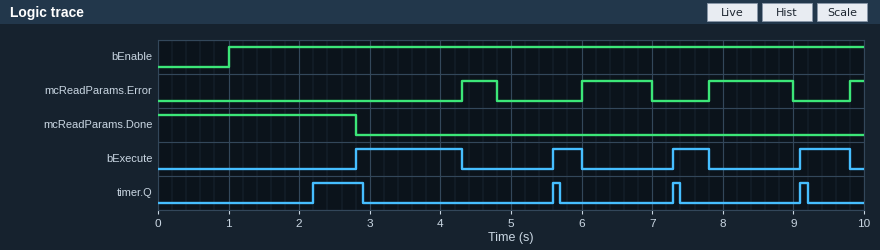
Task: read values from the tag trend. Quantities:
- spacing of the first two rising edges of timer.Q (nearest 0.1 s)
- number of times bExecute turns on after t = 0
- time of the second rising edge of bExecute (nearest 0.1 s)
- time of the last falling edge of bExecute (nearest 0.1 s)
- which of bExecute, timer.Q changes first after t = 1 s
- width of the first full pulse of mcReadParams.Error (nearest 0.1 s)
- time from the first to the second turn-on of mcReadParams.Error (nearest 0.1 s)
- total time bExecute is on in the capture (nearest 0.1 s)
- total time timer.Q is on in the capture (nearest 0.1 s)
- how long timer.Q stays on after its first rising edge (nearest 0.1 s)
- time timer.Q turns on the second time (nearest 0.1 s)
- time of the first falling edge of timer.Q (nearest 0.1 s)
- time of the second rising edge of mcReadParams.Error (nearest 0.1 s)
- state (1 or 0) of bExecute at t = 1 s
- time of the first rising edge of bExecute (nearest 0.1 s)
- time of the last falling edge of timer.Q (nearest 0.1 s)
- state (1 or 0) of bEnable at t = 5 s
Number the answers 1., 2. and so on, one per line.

1. 3.4 s
2. 4
3. 5.6 s
4. 9.8 s
5. timer.Q
6. 0.5 s
7. 1.7 s
8. 3.1 s
9. 1.0 s
10. 0.7 s
11. 5.6 s
12. 2.9 s
13. 6.0 s
14. 0
15. 2.8 s
16. 9.2 s
17. 1
